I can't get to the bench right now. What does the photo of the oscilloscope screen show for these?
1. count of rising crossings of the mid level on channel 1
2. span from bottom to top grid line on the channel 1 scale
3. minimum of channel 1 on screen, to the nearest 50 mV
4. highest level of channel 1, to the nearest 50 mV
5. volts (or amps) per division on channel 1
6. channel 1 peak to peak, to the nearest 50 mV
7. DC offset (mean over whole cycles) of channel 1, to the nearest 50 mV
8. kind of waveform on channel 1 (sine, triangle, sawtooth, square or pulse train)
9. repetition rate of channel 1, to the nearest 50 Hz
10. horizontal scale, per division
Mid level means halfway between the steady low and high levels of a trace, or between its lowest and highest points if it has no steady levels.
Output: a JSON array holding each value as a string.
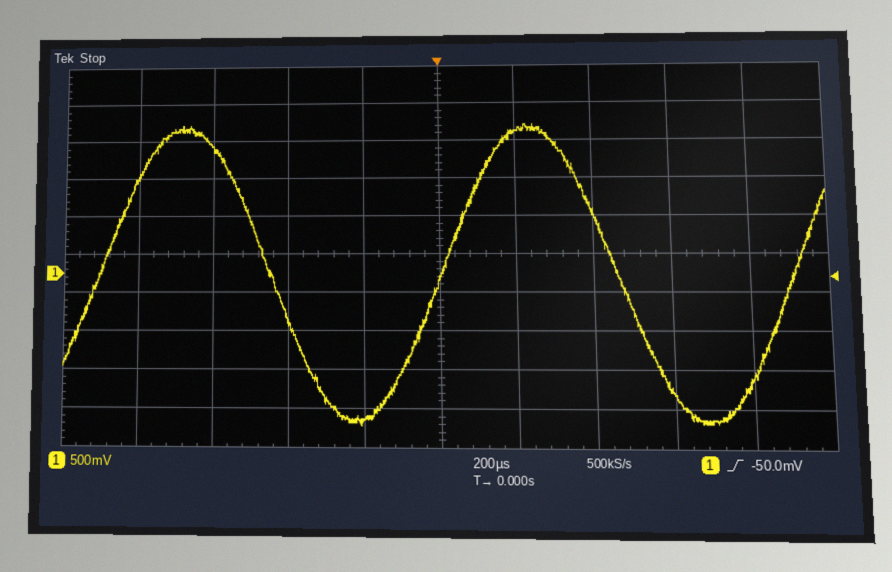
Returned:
["3", "5 V", "-1.95 V", "1.95 V", "500 mV", "3.90 V", "0 mV", "sine", "1.10 kHz", "200 µs"]
